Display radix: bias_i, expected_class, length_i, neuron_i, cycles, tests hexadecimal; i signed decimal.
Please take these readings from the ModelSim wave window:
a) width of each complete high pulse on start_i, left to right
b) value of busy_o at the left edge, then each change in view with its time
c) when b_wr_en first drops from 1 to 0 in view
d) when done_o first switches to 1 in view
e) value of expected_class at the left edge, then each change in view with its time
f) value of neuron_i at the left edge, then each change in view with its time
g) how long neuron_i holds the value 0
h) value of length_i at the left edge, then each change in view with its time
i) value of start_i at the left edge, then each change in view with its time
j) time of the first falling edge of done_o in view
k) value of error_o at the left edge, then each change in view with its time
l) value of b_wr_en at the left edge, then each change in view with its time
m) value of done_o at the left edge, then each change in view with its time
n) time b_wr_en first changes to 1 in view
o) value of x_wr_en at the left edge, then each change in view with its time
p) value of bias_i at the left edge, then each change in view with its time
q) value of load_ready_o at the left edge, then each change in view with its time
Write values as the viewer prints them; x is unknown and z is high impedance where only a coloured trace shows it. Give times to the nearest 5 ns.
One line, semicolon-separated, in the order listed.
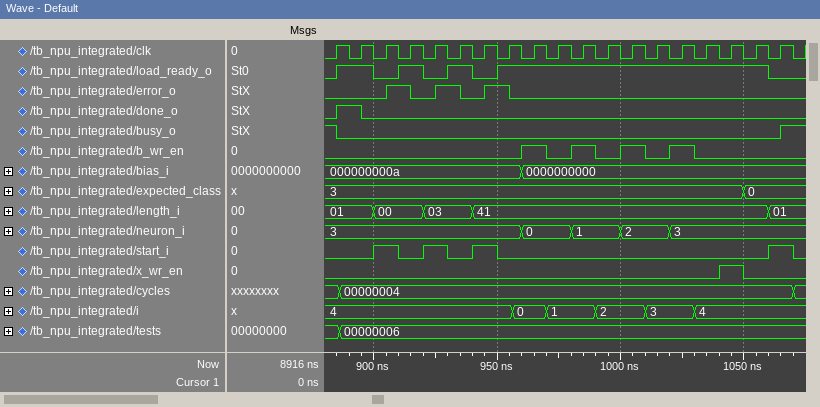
10 ns, 10 ns, 10 ns, 10 ns; 1, 0 at 885 ns, 1 at 1065 ns; 970 ns; 885 ns; 3, 0 at 1050 ns; 3, 0 at 960 ns, 1 at 980 ns, 2 at 1000 ns, 3 at 1020 ns; 20 ns; 01, 00 at 900 ns, 03 at 920 ns, 41 at 940 ns, 01 at 1060 ns; 0, 1 at 900 ns, 0 at 910 ns, 1 at 920 ns, 0 at 930 ns, 1 at 940 ns, 0 at 950 ns, 1 at 1060 ns, 0 at 1070 ns; 895 ns; 0, 1 at 905 ns, 0 at 915 ns, 1 at 925 ns, 0 at 935 ns, 1 at 945 ns, 0 at 955 ns; 0, 1 at 960 ns, 0 at 970 ns, 1 at 980 ns, 0 at 990 ns, 1 at 1000 ns, 0 at 1010 ns, 1 at 1020 ns, 0 at 1030 ns; 0, 1 at 885 ns, 0 at 895 ns; 960 ns; 0, 1 at 1040 ns, 0 at 1050 ns; 000000000a, 0000000000 at 960 ns; 0, 1 at 885 ns, 0 at 900 ns, 1 at 910 ns, 0 at 920 ns, 1 at 930 ns, 0 at 940 ns, 1 at 950 ns, 0 at 1060 ns
